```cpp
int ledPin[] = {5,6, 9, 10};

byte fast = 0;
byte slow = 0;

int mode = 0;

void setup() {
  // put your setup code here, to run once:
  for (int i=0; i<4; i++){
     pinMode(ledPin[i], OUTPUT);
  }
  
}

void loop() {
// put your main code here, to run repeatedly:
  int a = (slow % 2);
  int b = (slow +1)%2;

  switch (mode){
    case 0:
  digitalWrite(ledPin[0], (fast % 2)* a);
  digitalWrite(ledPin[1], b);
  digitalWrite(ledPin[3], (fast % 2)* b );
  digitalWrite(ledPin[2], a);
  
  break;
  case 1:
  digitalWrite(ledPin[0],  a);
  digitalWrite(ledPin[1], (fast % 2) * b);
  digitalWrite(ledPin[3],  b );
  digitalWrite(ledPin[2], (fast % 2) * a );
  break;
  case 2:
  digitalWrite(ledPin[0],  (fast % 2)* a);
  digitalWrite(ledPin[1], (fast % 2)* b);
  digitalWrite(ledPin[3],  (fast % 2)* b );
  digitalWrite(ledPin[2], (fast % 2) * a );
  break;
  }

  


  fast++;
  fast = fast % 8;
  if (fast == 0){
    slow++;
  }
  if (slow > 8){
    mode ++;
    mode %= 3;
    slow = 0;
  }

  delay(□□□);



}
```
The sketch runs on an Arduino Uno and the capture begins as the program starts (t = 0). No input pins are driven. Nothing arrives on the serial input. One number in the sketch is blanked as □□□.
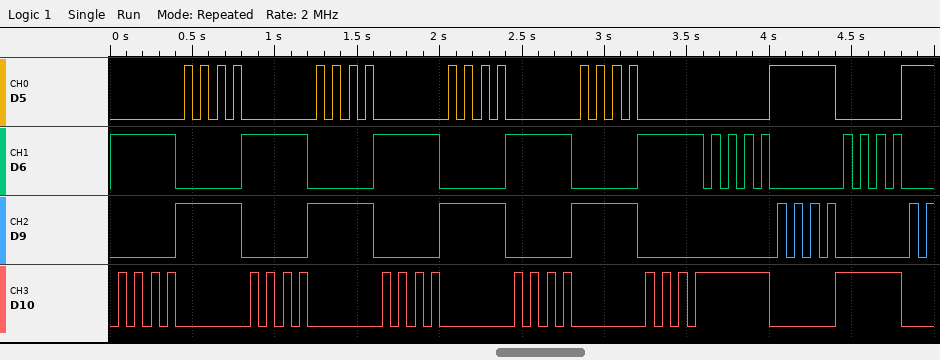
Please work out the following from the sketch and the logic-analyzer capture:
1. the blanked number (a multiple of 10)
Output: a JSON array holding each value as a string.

["50"]
